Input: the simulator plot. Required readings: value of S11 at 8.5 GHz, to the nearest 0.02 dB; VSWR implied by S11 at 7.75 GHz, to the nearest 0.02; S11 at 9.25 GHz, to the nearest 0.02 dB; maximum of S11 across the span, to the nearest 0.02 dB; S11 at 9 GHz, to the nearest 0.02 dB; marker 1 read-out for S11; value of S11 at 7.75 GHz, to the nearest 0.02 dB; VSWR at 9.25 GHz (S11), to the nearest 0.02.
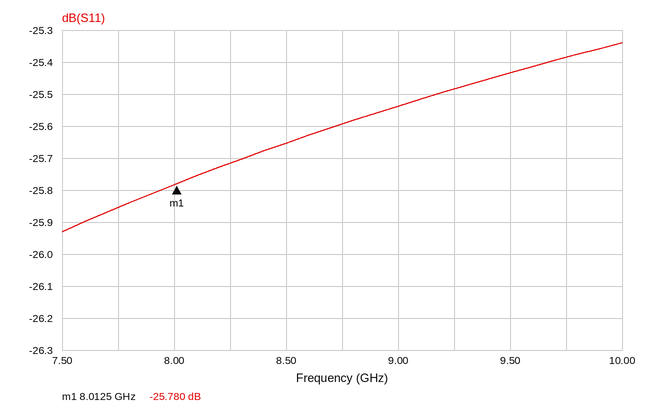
-25.66 dB
1.10
-25.48 dB
-25.34 dB
-25.54 dB
-25.780 dB
-25.86 dB
1.12
